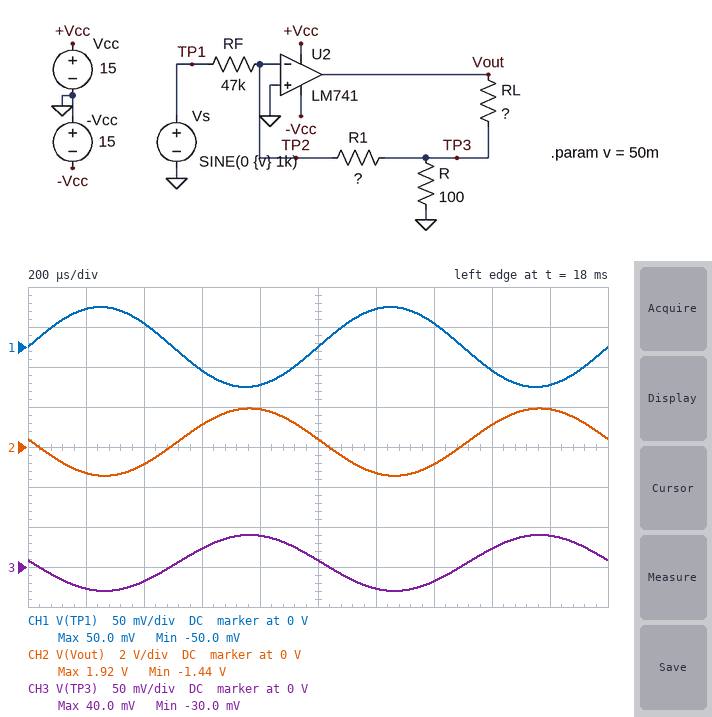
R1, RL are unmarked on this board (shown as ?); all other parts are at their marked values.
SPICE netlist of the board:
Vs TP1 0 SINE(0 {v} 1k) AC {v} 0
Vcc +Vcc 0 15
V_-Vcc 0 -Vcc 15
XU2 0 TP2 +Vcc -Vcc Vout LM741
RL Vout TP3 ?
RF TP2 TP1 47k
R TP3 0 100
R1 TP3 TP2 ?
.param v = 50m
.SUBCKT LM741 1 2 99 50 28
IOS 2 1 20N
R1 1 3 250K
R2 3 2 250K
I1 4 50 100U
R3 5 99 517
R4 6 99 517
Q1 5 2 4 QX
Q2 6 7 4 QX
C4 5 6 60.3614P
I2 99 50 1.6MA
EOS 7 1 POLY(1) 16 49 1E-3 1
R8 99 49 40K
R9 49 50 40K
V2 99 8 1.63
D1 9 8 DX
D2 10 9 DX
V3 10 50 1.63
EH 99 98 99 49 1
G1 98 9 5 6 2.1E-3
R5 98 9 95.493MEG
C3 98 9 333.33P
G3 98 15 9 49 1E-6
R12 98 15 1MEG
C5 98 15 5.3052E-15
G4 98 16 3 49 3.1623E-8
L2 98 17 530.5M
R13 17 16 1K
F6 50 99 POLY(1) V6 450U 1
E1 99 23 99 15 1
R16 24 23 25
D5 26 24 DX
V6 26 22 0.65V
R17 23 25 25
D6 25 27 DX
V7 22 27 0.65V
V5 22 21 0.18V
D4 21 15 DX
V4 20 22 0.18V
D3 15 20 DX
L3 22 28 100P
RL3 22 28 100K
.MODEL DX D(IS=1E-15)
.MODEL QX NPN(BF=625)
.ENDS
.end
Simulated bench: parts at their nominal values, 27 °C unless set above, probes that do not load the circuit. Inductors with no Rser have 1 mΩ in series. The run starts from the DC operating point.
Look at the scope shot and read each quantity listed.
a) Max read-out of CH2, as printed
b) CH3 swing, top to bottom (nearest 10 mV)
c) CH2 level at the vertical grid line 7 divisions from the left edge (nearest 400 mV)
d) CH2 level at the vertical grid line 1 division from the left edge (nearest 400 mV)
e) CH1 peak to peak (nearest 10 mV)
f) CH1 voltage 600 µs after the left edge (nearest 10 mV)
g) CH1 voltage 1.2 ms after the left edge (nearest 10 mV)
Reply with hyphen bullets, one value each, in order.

- 1.92 V
- 70 mV
- -800 mV
- -1.2 V
- 100 mV
- -30 mV
- 50 mV
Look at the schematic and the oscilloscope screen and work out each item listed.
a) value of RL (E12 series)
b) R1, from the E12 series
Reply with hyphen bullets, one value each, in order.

- 4.7 kΩ
- 33 kΩ
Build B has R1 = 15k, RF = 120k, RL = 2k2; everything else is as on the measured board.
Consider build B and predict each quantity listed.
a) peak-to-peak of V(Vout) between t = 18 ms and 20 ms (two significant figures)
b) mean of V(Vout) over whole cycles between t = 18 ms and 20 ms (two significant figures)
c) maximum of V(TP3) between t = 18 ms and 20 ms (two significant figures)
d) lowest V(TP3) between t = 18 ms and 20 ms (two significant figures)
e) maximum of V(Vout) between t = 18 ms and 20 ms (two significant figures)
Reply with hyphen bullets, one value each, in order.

- 290 mV
- 61 mV
- 8.9 mV
- -3.6 mV
- 210 mV
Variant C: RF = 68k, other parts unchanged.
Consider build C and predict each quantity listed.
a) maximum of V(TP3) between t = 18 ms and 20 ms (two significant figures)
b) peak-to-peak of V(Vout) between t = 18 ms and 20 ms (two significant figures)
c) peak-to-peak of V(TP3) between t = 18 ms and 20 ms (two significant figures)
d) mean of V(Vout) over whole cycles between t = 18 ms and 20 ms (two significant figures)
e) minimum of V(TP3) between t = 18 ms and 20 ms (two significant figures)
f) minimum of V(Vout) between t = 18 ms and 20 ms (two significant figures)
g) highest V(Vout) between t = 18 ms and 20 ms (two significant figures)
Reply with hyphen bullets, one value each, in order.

- 29 mV
- 2.3 V
- 48 mV
- 230 mV
- -19 mV
- -930 mV
- 1.4 V
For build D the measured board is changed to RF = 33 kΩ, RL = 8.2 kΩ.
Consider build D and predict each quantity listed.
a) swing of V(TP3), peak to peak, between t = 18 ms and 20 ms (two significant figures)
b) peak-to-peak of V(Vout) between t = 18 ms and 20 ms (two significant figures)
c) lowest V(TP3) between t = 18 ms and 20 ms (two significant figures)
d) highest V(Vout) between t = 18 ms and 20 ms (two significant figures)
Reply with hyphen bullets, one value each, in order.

- 98 mV
- 8.2 V
- -44 mV
- 4.5 V
